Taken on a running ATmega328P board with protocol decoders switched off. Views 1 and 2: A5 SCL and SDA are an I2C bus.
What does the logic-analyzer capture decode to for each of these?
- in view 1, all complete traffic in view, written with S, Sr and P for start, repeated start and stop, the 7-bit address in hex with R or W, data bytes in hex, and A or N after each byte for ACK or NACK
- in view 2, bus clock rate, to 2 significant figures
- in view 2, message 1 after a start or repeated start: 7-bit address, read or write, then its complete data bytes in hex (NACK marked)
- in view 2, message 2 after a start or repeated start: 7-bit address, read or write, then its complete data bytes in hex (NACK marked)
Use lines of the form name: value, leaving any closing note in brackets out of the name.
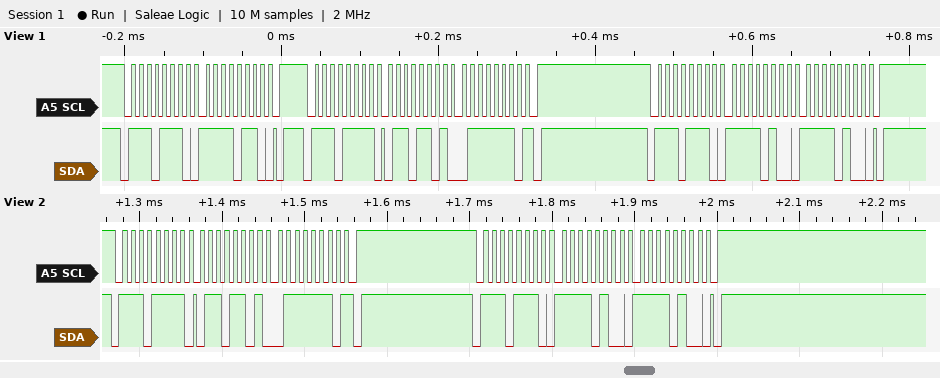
in view 1, all complete traffic in view, written with S, Sr and P for start, repeated start and stop, the 7-bit address in hex with R or W, data bytes in hex, and A or N after each byte for ACK or NACK: S 77W A F6 A P S 77R A 6D A 7E N P S 77W A F4 A F4 A P
in view 2, bus clock rate, to 2 significant figures: 100 kHz
in view 2, message 1 after a start or repeated start: 7-bit address, read or write, then its complete data bytes in hex: 0x77 read: 6D 7E NACK
in view 2, message 2 after a start or repeated start: 7-bit address, read or write, then its complete data bytes in hex: 0x77 write: F4 F4
